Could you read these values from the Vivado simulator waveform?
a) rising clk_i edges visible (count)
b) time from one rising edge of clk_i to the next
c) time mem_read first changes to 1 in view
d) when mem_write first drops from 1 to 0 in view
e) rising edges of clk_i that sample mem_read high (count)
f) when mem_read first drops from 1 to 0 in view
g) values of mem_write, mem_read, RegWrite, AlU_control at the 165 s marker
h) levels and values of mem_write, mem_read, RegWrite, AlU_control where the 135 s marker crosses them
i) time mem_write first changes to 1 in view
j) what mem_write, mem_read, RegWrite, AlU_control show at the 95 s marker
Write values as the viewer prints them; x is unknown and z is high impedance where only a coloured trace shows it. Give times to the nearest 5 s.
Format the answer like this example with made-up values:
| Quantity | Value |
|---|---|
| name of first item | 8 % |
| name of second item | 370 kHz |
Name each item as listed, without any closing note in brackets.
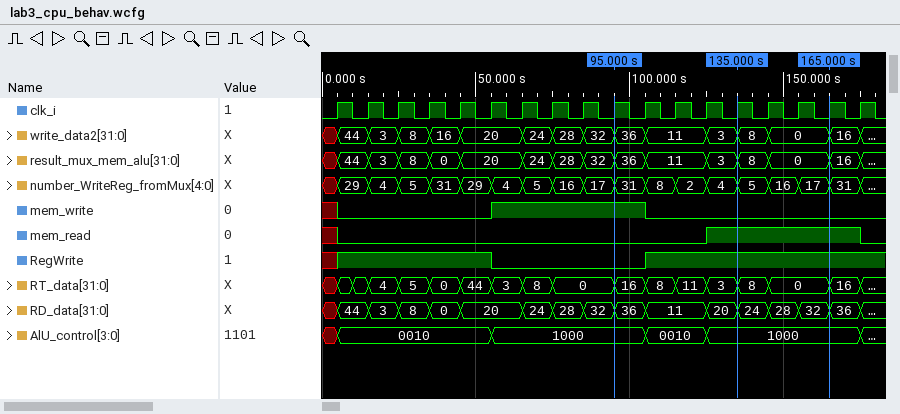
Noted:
| Quantity | Value |
|---|---|
| rising clk_i edges visible | 18 |
| time from one rising edge of clk_i to the next | 10 s |
| time mem_read first changes to 1 in view | 125 s |
| when mem_write first drops from 1 to 0 in view | 105 s |
| rising edges of clk_i that sample mem_read high | 5 |
| when mem_read first drops from 1 to 0 in view | 175 s |
| values of mem_write, mem_read, RegWrite, AlU_control at the 165 s marker | mem_write=0, mem_read=1, RegWrite=1, AlU_control=1000 |
| levels and values of mem_write, mem_read, RegWrite, AlU_control where the 135 s marker crosses them | mem_write=0, mem_read=1, RegWrite=1, AlU_control=1000 |
| time mem_write first changes to 1 in view | 55 s |
| what mem_write, mem_read, RegWrite, AlU_control show at the 95 s marker | mem_write=1, mem_read=0, RegWrite=0, AlU_control=1000 |
